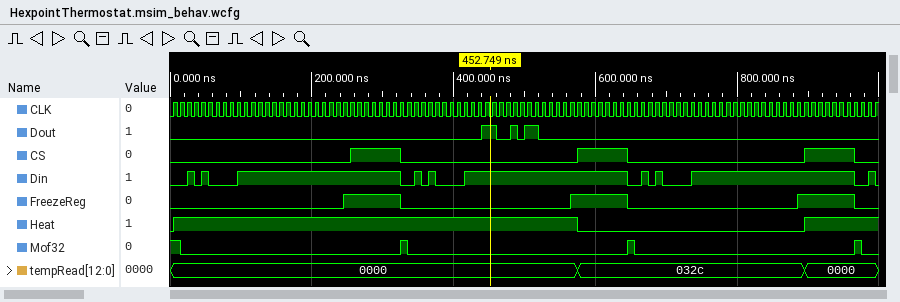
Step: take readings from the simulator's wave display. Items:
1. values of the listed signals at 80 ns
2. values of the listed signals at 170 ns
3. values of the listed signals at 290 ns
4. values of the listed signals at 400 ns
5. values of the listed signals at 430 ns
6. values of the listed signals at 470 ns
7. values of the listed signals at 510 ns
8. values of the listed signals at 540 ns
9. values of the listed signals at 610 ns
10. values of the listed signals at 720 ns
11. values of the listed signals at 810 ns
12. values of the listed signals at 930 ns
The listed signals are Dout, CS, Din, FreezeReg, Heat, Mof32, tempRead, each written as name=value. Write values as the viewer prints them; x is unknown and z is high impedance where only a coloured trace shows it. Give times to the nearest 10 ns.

Dout=0, CS=0, Din=0, FreezeReg=0, Heat=1, Mof32=0, tempRead=0000
Dout=0, CS=0, Din=1, FreezeReg=0, Heat=1, Mof32=0, tempRead=0000
Dout=0, CS=1, Din=1, FreezeReg=1, Heat=1, Mof32=0, tempRead=0000
Dout=0, CS=0, Din=0, FreezeReg=0, Heat=1, Mof32=0, tempRead=0000
Dout=0, CS=0, Din=1, FreezeReg=0, Heat=1, Mof32=0, tempRead=0000
Dout=0, CS=0, Din=1, FreezeReg=0, Heat=1, Mof32=0, tempRead=0000
Dout=1, CS=0, Din=1, FreezeReg=0, Heat=1, Mof32=0, tempRead=0000
Dout=0, CS=0, Din=1, FreezeReg=0, Heat=1, Mof32=0, tempRead=0000
Dout=0, CS=1, Din=1, FreezeReg=1, Heat=0, Mof32=0, tempRead=032c
Dout=0, CS=0, Din=0, FreezeReg=0, Heat=0, Mof32=0, tempRead=032c
Dout=0, CS=0, Din=1, FreezeReg=0, Heat=0, Mof32=0, tempRead=032c
Dout=0, CS=1, Din=1, FreezeReg=1, Heat=1, Mof32=0, tempRead=0000
